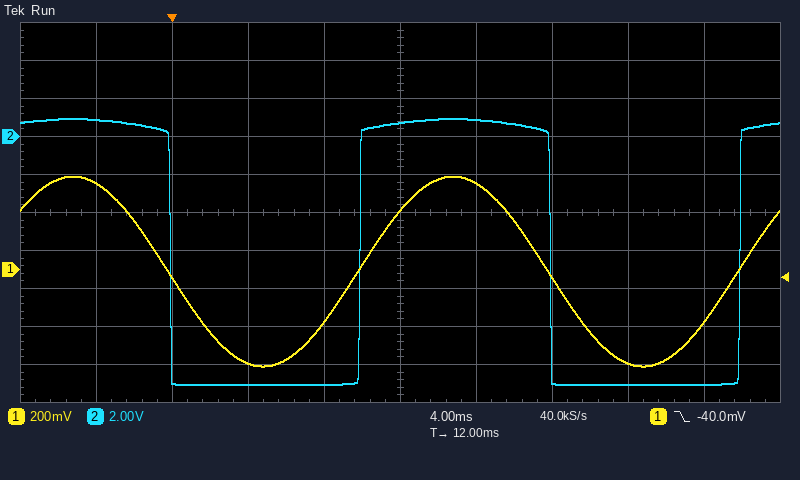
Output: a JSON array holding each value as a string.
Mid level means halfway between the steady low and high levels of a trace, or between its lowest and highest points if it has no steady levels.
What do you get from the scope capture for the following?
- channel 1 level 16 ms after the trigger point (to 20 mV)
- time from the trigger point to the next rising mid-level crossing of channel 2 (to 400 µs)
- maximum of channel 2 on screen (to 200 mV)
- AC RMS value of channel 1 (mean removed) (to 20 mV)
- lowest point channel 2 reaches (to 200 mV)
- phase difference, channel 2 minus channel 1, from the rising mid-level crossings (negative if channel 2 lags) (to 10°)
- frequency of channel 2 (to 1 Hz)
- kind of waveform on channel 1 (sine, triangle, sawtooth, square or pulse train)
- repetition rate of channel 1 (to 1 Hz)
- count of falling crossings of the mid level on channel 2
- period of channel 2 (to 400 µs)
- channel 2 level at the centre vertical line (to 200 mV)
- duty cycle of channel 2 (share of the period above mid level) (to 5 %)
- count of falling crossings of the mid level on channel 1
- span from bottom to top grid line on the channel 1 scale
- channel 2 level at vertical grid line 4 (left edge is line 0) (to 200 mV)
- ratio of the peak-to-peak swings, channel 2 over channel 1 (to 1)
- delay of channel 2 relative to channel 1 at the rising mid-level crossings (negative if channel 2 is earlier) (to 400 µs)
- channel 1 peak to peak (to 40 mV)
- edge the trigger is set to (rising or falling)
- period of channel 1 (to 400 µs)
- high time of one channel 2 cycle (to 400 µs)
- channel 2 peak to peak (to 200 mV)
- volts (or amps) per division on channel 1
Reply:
["460 mV", "10.0 ms", "1.0 V", "360 mV", "-13.0 V", "0°", "50 Hz", "sine", "50 Hz", "2", "20.0 ms", "800 mV", "50 %", "2", "2 V", "-13.0 V", "14", "0.0 ms", "1.00 V", "falling", "20.0 ms", "10.0 ms", "14.0 V", "200 mV"]
